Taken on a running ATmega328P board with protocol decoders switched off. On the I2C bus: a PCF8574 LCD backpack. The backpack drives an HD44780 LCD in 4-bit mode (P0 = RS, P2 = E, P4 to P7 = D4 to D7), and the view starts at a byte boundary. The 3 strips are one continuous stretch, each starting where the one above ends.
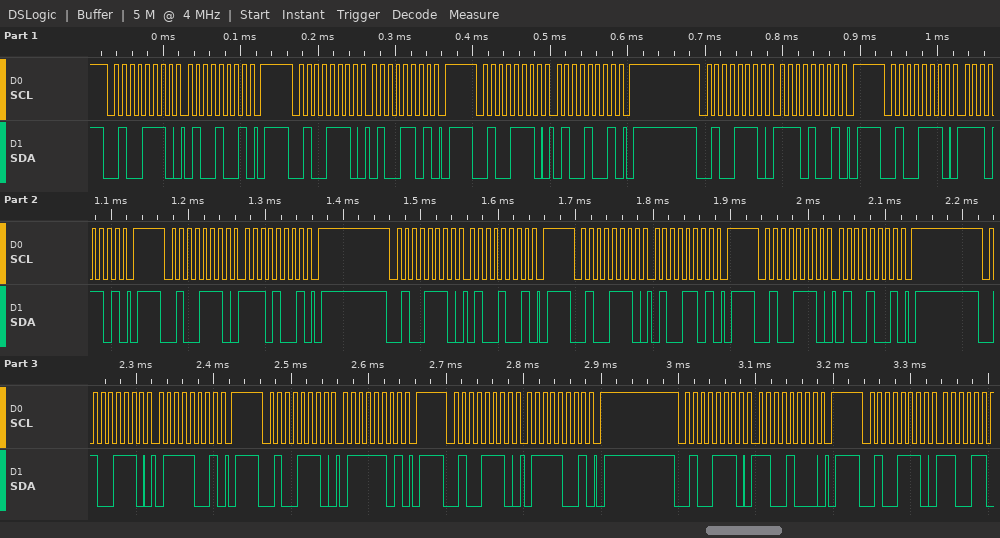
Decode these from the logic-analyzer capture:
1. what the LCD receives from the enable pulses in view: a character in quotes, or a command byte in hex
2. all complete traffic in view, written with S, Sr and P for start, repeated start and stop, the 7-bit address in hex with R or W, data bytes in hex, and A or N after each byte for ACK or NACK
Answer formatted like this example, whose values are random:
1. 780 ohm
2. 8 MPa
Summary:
1. 'N' 'G'
2. S 27W A 49 A P S 27W A 4D A P S 27W A 49 A P S 27W A E9 A P S 27W A ED A P S 27W A E9 A P S 27W A 49 A P S 27W A 4D A P S 27W A 49 A P S 27W A 79 A P S 27W A 7D A P S 27W A 79 A P S 27W A C8 A P S 27W A
